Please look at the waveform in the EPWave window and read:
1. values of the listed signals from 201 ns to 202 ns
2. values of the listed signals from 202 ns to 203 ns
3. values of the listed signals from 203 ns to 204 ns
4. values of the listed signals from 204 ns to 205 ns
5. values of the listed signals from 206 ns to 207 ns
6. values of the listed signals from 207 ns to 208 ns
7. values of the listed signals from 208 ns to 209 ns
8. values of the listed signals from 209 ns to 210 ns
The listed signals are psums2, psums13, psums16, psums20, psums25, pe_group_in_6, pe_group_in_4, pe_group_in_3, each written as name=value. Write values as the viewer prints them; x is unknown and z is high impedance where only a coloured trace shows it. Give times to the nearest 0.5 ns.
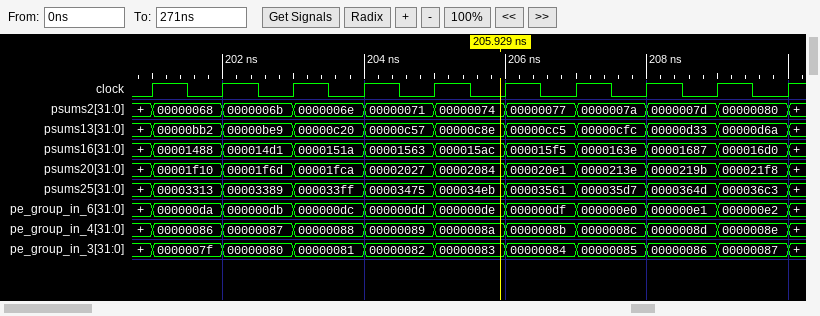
psums2=00000068, psums13=00000bb2, psums16=00001488, psums20=00001f10, psums25=00003313, pe_group_in_6=000000da, pe_group_in_4=00000086, pe_group_in_3=0000007f
psums2=0000006b, psums13=00000be9, psums16=000014d1, psums20=00001f6d, psums25=00003389, pe_group_in_6=000000db, pe_group_in_4=00000087, pe_group_in_3=00000080
psums2=0000006e, psums13=00000c20, psums16=0000151a, psums20=00001fca, psums25=000033ff, pe_group_in_6=000000dc, pe_group_in_4=00000088, pe_group_in_3=00000081
psums2=00000071, psums13=00000c57, psums16=00001563, psums20=00002027, psums25=00003475, pe_group_in_6=000000dd, pe_group_in_4=00000089, pe_group_in_3=00000082
psums2=00000077, psums13=00000cc5, psums16=000015f5, psums20=000020e1, psums25=00003561, pe_group_in_6=000000df, pe_group_in_4=0000008b, pe_group_in_3=00000084
psums2=0000007a, psums13=00000cfc, psums16=0000163e, psums20=0000213e, psums25=000035d7, pe_group_in_6=000000e0, pe_group_in_4=0000008c, pe_group_in_3=00000085
psums2=0000007d, psums13=00000d33, psums16=00001687, psums20=0000219b, psums25=0000364d, pe_group_in_6=000000e1, pe_group_in_4=0000008d, pe_group_in_3=00000086
psums2=00000080, psums13=00000d6a, psums16=000016d0, psums20=000021f8, psums25=000036c3, pe_group_in_6=000000e2, pe_group_in_4=0000008e, pe_group_in_3=00000087
